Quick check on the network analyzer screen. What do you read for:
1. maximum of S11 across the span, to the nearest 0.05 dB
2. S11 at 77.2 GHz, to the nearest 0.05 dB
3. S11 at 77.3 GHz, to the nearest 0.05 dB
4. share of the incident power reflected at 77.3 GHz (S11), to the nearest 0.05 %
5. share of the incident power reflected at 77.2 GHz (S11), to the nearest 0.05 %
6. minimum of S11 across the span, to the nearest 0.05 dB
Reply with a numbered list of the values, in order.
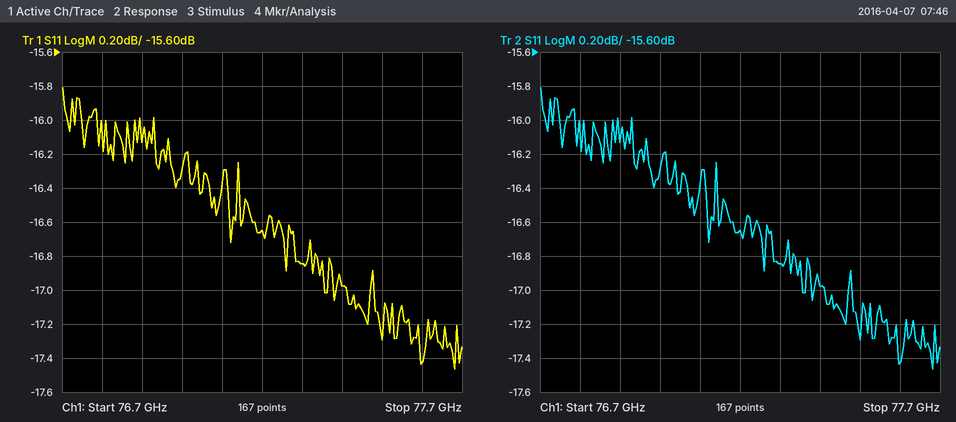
1. -15.80 dB
2. -16.65 dB
3. -16.85 dB
4. 2.05 %
5. 2.15 %
6. -17.45 dB
